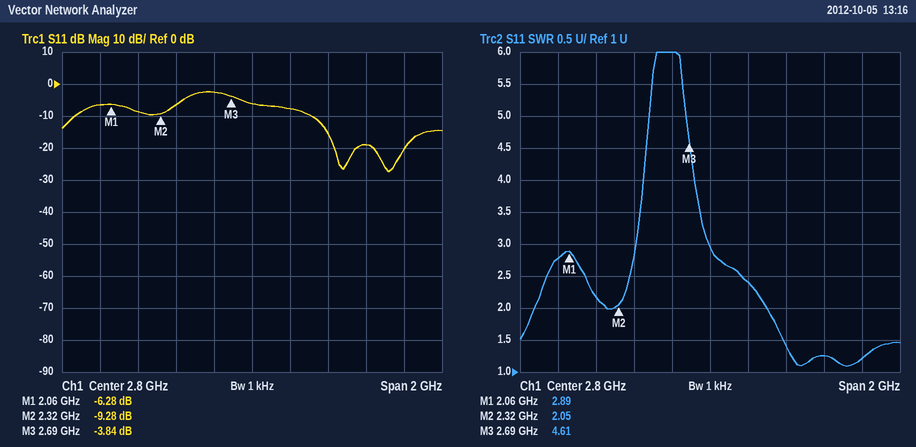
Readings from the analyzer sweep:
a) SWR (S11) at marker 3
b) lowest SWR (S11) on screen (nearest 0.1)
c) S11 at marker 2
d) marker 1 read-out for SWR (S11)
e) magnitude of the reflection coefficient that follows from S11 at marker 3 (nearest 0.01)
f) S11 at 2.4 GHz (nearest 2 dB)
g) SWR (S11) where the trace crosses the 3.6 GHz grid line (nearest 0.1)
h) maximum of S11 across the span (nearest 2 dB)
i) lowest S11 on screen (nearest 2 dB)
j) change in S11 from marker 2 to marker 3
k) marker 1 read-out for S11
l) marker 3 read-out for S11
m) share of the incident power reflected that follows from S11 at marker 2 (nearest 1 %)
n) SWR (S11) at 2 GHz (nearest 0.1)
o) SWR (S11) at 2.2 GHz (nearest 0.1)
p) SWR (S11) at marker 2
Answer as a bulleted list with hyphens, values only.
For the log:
- 4.61
- 1.1
- -9.28 dB
- 2.89
- 0.64
- -6 dB
- 1.2
- -2 dB
- -28 dB
- 5.44 dB
- -6.28 dB
- -3.84 dB
- 12 %
- 2.8
- 2.2
- 2.05
